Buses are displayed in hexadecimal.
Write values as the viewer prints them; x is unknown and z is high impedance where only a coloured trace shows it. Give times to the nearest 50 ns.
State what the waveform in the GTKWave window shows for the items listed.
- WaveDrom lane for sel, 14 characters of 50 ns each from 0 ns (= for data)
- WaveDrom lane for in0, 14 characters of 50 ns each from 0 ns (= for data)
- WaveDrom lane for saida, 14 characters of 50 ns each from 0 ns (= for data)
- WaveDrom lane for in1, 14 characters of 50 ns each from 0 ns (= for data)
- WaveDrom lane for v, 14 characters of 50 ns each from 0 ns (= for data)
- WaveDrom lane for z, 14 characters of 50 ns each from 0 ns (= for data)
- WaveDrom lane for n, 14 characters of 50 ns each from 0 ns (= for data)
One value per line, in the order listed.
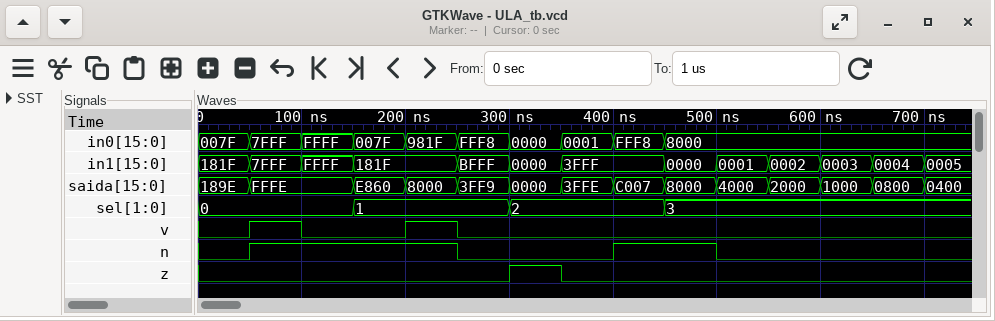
{name: 'sel', wave: '=..=..=..=....', data: '0 1 2 3'}
{name: 'in0', wave: '==========....', data: '007F 7FFF FFFF 007F 981F FFF8 0000 0001 FFF8 8000'}
{name: 'saida', wave: '==.===========', data: '189E FFFE E860 8000 3FF9 0000 3FFE C007 8000 4000 2000 1000 0800'}
{name: 'in1', wave: '====.===.=====', data: '181F 7FFF FFFF 181F BFFF 0000 3FFF 0000 0001 0002 0003 0004'}
{name: 'v', wave: '010.10........'}
{name: 'z', wave: '0.....10......'}
{name: 'n', wave: '01...0..1.0...'}
